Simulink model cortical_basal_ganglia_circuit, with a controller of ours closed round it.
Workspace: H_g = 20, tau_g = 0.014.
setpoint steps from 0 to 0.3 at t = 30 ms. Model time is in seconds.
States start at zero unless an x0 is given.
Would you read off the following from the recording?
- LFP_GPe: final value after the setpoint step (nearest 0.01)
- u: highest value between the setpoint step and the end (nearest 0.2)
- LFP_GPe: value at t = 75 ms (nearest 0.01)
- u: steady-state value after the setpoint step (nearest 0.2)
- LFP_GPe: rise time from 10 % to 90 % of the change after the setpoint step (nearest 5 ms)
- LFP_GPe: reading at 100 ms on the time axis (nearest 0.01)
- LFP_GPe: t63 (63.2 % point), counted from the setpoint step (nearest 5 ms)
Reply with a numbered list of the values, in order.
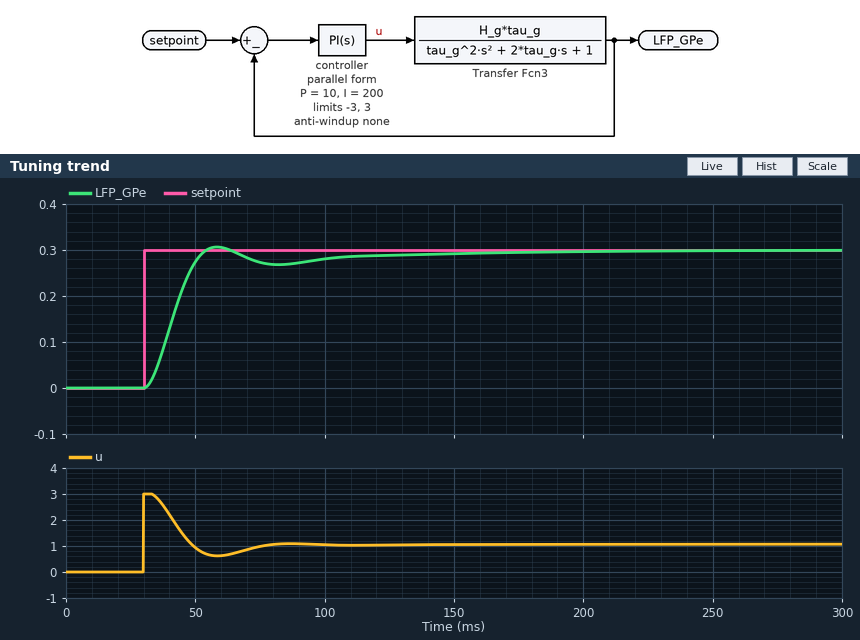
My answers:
1. 0.30
2. 3.0
3. 0.27
4. 1.0
5. 15 ms
6. 0.28
7. 15 ms
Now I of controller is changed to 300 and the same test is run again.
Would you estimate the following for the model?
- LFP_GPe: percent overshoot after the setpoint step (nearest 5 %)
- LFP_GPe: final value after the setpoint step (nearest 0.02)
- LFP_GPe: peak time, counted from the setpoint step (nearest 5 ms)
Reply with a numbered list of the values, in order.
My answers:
1. 10 %
2. 0.30
3. 30 ms
